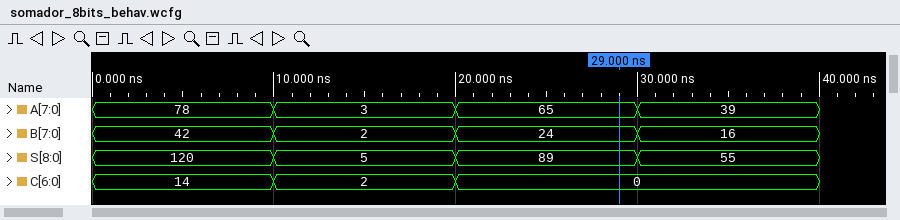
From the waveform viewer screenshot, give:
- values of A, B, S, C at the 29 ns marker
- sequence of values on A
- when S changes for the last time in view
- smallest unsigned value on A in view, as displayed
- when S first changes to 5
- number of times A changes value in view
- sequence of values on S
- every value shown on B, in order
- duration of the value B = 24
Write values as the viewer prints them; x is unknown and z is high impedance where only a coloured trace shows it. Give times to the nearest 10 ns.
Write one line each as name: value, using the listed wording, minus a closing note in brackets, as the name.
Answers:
values of A, B, S, C at the 29 ns marker: A=65, B=24, S=89, C=0
sequence of values on A: 78, 3, 65, 39
when S changes for the last time in view: 30 ns
smallest unsigned value on A in view, as displayed: 3
when S first changes to 5: 10 ns
number of times A changes value in view: 3
sequence of values on S: 120, 5, 89, 55
every value shown on B, in order: 42, 2, 24, 16
duration of the value B = 24: 10 ns
